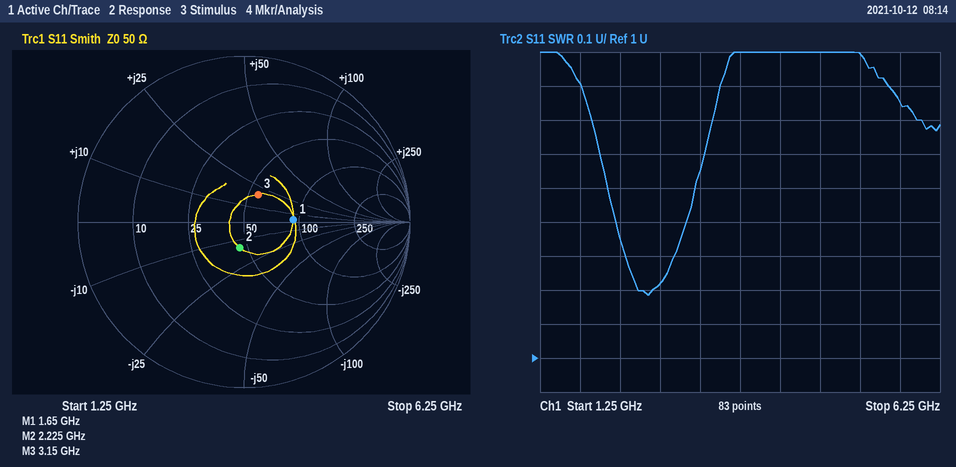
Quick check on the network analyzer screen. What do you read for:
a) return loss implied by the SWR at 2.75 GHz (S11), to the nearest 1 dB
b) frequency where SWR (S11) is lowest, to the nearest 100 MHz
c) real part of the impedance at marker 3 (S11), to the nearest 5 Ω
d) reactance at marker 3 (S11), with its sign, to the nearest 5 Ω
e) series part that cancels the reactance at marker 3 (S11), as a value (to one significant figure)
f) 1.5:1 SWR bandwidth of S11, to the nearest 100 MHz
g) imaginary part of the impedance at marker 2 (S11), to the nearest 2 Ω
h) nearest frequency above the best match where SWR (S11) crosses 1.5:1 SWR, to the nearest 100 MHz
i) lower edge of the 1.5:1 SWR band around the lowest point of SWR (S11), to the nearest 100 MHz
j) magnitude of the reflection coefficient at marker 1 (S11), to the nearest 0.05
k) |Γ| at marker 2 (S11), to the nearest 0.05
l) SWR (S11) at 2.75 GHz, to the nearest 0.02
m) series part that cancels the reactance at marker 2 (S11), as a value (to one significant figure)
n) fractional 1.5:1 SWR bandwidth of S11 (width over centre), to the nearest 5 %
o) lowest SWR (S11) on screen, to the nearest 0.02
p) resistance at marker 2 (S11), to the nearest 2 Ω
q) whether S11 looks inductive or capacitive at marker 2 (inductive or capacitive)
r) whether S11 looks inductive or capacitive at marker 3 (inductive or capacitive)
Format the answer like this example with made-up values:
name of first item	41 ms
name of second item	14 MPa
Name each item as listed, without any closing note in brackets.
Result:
return loss implied by the SWR at 2.75 GHz (S11), to the nearest 1 dB	20 dB
frequency where SWR (S11) is lowest, to the nearest 100 MHz	2.6 GHz
real part of the impedance at marker 3 (S11), to the nearest 5 Ω	55 Ω
reactance at marker 3 (S11), with its sign, to the nearest 5 Ω	+20 Ω
series part that cancels the reactance at marker 3 (S11), as a value	3 pF
1.5:1 SWR bandwidth of S11, to the nearest 100 MHz	1.1 GHz
imaginary part of the impedance at marker 2 (S11), to the nearest 2 Ω	-14 Ω
nearest frequency above the best match where SWR (S11) crosses 1.5:1 SWR, to the nearest 100 MHz	3.2 GHz
lower edge of the 1.5:1 SWR band around the lowest point of SWR (S11), to the nearest 100 MHz	2.1 GHz
magnitude of the reflection coefficient at marker 1 (S11), to the nearest 0.05	0.30
|Γ| at marker 2 (S11), to the nearest 0.05	0.15
SWR (S11) at 2.75 GHz, to the nearest 0.02	1.22
series part that cancels the reactance at marker 2 (S11), as a value	1 nH
fractional 1.5:1 SWR bandwidth of S11 (width over centre), to the nearest 5 %	40 %
lowest SWR (S11) on screen, to the nearest 0.02	1.18
resistance at marker 2 (S11), to the nearest 2 Ω	46 Ω
whether S11 looks inductive or capacitive at marker 2	capacitive
whether S11 looks inductive or capacitive at marker 3	inductive
